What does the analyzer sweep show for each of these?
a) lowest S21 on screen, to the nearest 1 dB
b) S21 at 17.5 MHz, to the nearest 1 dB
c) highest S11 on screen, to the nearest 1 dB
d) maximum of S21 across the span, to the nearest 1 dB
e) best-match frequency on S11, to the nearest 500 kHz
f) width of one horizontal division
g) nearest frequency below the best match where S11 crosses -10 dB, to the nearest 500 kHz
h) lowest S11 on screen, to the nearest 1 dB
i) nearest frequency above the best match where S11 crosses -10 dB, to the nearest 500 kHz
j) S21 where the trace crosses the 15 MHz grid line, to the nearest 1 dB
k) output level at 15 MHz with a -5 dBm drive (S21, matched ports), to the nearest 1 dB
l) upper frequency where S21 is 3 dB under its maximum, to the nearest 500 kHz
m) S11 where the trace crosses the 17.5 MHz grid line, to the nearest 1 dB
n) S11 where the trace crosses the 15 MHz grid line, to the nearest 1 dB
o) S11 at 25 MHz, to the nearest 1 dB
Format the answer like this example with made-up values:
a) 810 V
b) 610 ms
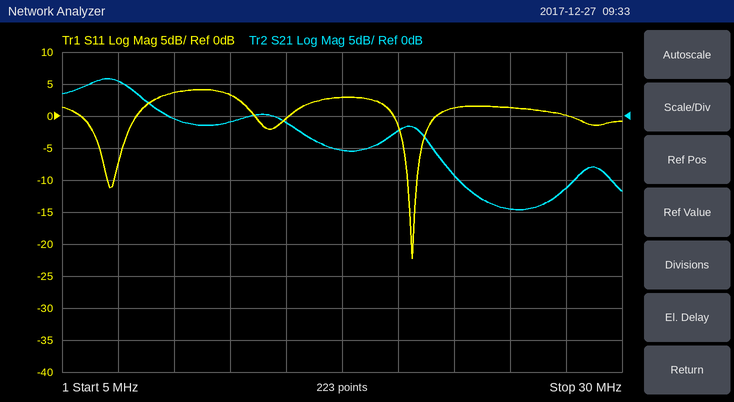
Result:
a) -15 dB
b) -5 dB
c) 4 dB
d) 6 dB
e) 20.5 MHz
f) 2.5 MHz
g) 20.5 MHz
h) -22 dB
i) 21.0 MHz
j) -1 dB
k) -6 dBm
l) 8.5 MHz
m) 3 dB
n) 0 dB
o) 1 dB
